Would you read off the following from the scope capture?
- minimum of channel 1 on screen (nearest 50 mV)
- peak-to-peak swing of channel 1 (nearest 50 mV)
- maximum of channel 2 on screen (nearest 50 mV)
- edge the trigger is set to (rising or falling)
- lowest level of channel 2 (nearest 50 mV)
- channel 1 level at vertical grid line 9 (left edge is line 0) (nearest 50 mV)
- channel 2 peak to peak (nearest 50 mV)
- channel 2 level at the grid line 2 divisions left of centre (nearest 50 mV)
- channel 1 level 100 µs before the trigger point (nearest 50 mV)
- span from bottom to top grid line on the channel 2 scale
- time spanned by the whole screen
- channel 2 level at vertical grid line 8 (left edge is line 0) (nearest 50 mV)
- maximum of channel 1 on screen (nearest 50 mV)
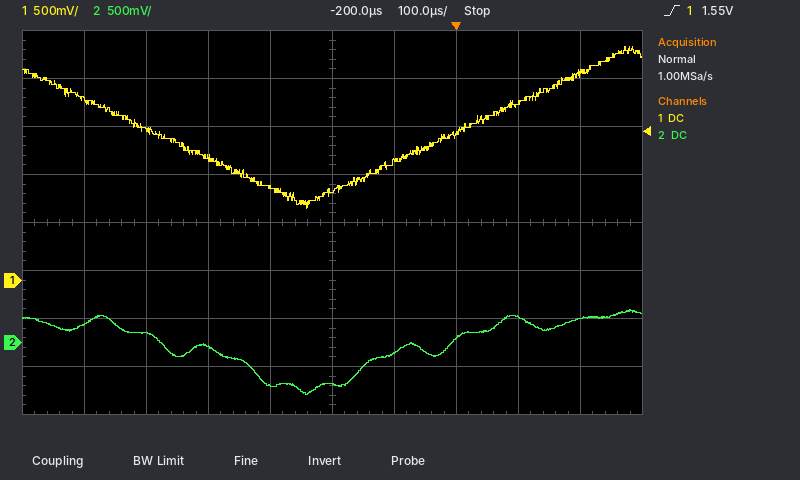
750 mV
1.70 V
350 mV
rising
-550 mV
2.15 V
900 mV
-50 mV
1.25 V
4 V
1 ms
250 mV
2.45 V
